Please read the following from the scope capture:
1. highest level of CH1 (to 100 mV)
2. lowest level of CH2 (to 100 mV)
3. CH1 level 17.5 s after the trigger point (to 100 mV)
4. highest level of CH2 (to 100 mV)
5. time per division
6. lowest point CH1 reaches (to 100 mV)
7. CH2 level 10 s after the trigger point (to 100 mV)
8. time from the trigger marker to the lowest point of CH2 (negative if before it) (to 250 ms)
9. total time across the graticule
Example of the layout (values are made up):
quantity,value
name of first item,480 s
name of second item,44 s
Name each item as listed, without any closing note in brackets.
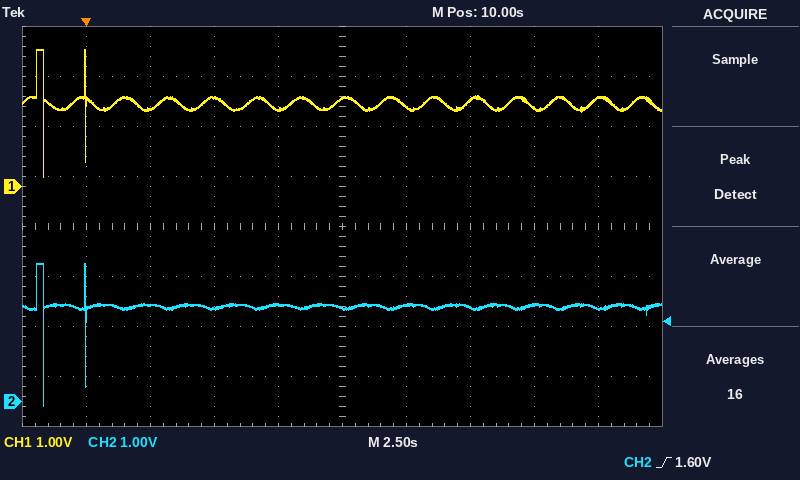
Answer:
quantity,value
highest level of CH1,2.7 V
lowest level of CH2,-100 mV
CH1 level 17.5 s after the trigger point,1.6 V
highest level of CH2,2.8 V
time per division,2.5 s
lowest point CH1 reaches,200 mV
CH2 level 10 s after the trigger point,1.9 V
time from the trigger marker to the lowest point of CH2 (negative if before it),-1.75 s
total time across the graticule,25 s
